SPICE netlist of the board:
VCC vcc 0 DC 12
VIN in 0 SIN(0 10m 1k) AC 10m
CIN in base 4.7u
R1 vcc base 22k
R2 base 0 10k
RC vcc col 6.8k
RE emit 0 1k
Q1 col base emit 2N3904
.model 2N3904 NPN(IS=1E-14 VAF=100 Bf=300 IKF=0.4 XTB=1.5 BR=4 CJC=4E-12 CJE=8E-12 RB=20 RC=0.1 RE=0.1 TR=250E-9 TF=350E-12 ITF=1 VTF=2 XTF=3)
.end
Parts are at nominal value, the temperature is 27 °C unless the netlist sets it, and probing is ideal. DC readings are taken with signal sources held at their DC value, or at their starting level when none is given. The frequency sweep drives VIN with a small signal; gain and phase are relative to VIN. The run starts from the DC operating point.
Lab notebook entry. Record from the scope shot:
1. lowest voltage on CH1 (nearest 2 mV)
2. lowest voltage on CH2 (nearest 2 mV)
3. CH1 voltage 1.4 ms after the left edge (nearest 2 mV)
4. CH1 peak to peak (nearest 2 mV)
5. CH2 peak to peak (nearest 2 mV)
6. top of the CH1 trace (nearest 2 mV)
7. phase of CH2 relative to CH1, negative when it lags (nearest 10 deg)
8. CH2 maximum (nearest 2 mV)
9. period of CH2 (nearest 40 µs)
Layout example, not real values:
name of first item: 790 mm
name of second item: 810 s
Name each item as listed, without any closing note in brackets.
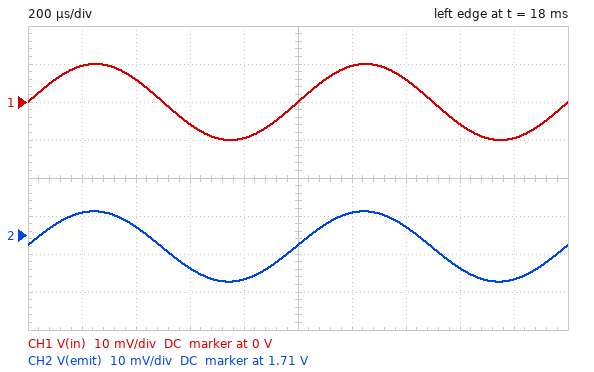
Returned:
lowest voltage on CH1: -10 mV
lowest voltage on CH2: 1.698 V
CH1 voltage 1.4 ms after the left edge: 6 mV
CH1 peak to peak: 20 mV
CH2 peak to peak: 18 mV
top of the CH1 trace: 10 mV
phase of CH2 relative to CH1, negative when it lags: 0 deg
CH2 maximum: 1.716 V
period of CH2: 1.00 ms
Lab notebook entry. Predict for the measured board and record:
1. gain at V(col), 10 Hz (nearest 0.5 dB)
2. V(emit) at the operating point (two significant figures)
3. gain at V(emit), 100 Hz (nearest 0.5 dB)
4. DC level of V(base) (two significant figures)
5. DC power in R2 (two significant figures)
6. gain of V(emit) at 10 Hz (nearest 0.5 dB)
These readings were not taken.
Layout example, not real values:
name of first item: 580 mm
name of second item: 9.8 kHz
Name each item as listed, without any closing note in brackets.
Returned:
gain at V(col), 10 Hz: -14.0 dB
V(emit) at the operating point: 1.7 V
gain at V(emit), 100 Hz: -1.5 dB
DC level of V(base): 2.4 V
DC power in R2: 570 µW
gain of V(emit) at 10 Hz: -13.0 dB
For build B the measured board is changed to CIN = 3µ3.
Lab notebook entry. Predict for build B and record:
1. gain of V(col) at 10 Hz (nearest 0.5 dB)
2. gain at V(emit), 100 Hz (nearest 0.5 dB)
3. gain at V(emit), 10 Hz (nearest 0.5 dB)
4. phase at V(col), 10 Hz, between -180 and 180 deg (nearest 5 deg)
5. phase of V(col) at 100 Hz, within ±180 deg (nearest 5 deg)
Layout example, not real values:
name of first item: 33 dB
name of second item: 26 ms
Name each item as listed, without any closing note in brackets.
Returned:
gain of V(col) at 10 Hz: -17.0 dB
gain at V(emit), 100 Hz: -2.0 dB
gain at V(emit), 10 Hz: -16.0 dB
phase at V(col), 10 Hz, between -180 and 180 deg: 80 deg
phase of V(col) at 100 Hz, within ±180 deg: 30 deg
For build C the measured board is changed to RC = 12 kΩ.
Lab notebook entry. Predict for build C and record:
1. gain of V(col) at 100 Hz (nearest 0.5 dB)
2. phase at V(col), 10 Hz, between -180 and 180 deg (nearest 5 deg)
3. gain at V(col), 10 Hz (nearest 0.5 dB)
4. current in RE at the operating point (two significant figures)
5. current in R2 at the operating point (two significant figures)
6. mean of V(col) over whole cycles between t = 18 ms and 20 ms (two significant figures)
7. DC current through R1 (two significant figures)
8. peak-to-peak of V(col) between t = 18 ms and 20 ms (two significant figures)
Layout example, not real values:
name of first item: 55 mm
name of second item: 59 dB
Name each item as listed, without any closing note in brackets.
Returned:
gain of V(col) at 100 Hz: -1.5 dB
phase at V(col), 10 Hz, between -180 and 180 deg: 75 deg
gain at V(col), 10 Hz: -13.0 dB
current in RE at the operating point: 1.2 mA
current in R2 at the operating point: 190 µA
mean of V(col) over whole cycles between t = 18 ms and 20 ms: 1.2 V
DC current through R1: 460 µA
peak-to-peak of V(col) between t = 18 ms and 20 ms: 18 mV
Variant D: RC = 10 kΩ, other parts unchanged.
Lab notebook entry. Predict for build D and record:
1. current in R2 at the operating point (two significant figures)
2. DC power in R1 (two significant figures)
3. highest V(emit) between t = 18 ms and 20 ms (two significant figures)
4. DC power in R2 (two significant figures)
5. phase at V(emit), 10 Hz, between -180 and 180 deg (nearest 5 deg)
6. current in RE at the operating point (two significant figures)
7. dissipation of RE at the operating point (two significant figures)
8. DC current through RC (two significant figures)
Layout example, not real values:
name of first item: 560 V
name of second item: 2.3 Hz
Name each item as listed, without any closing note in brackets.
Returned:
current in R2 at the operating point: 200 µA
DC power in R1: 4.5 mW
highest V(emit) between t = 18 ms and 20 ms: 1.3 V
DC power in R2: 400 µW
phase at V(emit), 10 Hz, between -180 and 180 deg: 75 deg
current in RE at the operating point: 1.3 mA
dissipation of RE at the operating point: 1.7 mW
DC current through RC: 1.1 mA
